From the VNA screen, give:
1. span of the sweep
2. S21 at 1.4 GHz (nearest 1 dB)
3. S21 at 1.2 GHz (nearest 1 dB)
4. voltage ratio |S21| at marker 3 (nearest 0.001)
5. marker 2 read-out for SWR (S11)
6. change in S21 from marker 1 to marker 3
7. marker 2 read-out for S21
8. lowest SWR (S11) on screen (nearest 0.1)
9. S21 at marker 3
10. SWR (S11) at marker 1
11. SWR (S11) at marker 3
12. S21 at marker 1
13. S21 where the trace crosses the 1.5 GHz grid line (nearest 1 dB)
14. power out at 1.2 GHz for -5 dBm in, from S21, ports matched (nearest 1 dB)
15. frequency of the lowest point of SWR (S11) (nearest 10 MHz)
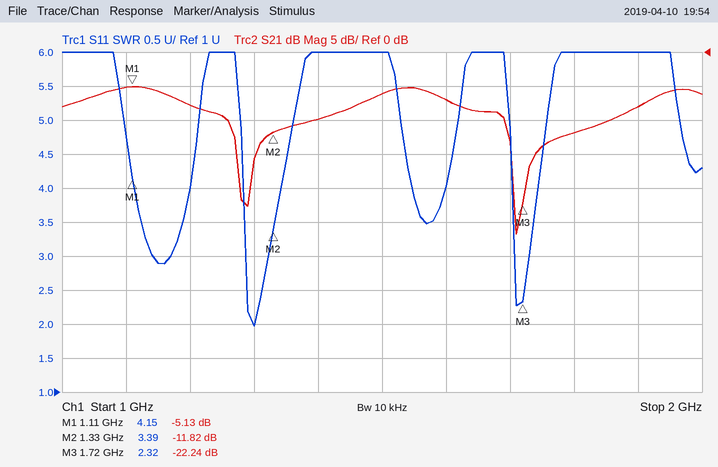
1 GHz
-10 dB
-8 dB
0.077
3.39
-17.11 dB
-11.82 dB
2.0
-22.24 dB
4.15
2.32
-5.13 dB
-6 dB
-13 dBm
1.30 GHz
